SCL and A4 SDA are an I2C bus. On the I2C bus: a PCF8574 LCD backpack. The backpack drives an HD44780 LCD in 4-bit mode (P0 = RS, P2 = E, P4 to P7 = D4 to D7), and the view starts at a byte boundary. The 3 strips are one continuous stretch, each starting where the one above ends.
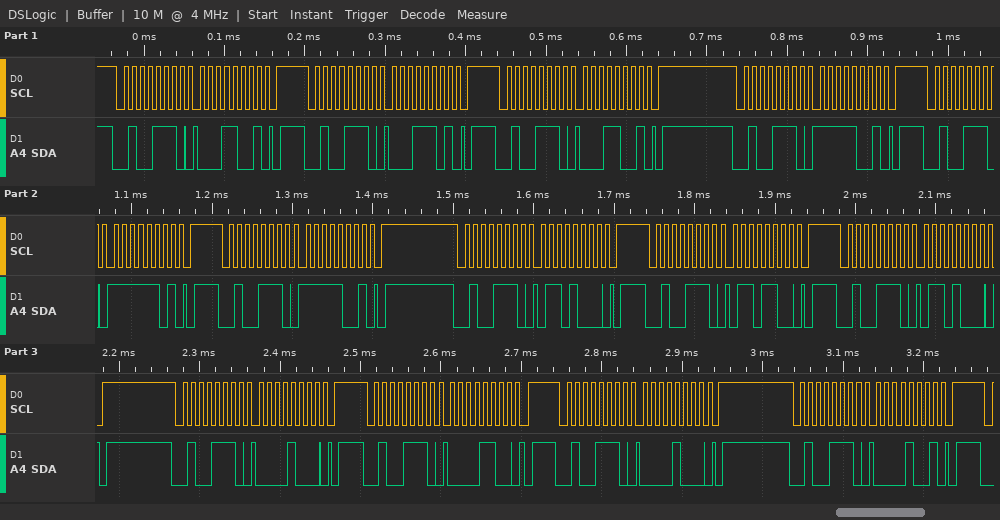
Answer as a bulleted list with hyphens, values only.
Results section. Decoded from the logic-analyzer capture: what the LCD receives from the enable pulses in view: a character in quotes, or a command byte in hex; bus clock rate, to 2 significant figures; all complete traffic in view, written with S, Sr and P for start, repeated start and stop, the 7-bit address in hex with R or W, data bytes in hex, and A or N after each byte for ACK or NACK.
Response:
- data 0x1F 0x60
- 100 kHz
- S 27W A 19 A P S 27W A 1D A P S 27W A 19 A P S 27W A F9 A P S 27W A FD A P S 27W A F9 A P S 27W A 68 A P S 27W A 6C A P S 27W A 68 A P S 27W A 08 A P S 27W A 0C A P S 27W A 08 A P S 27W A 09 A P
